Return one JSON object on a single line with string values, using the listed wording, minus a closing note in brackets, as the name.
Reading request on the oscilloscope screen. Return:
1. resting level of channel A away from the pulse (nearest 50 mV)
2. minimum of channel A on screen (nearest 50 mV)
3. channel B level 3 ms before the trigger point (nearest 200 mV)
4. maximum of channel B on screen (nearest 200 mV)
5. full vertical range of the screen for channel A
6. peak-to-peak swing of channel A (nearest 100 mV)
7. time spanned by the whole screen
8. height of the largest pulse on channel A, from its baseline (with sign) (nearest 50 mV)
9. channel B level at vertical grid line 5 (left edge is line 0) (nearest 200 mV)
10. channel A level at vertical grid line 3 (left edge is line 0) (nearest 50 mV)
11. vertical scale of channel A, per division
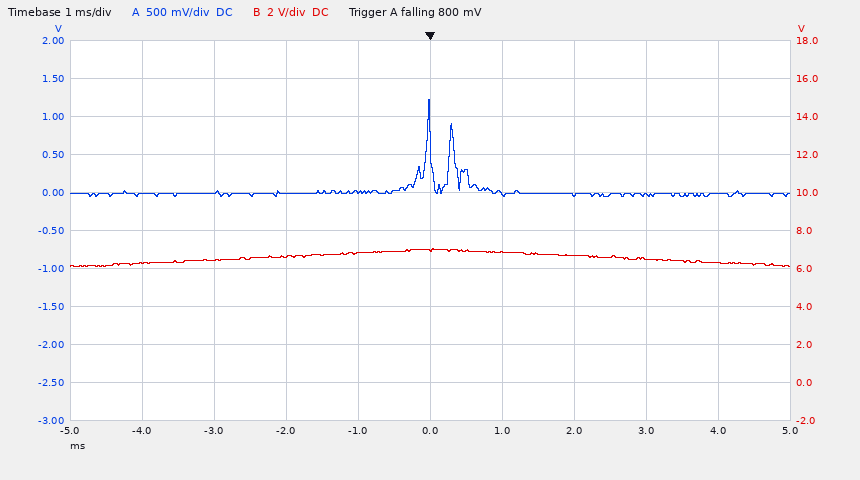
{"resting level of channel A away from the pulse": "0 mV", "minimum of channel A on screen": "-50 mV", "channel B level 3 ms before the trigger point": "6.4 V", "maximum of channel B on screen": "7.0 V", "full vertical range of the screen for channel A": "5 V", "peak-to-peak swing of channel A": "1.30 V", "time spanned by the whole screen": "10 ms", "height of the largest pulse on channel A, from its baseline (with sign)": "+1.25 V", "channel B level at vertical grid line 5 (left edge is line 0)": "7.0 V", "channel A level at vertical grid line 3 (left edge is line 0)": "0 mV", "vertical scale of channel A, per division": "500 mV"}
